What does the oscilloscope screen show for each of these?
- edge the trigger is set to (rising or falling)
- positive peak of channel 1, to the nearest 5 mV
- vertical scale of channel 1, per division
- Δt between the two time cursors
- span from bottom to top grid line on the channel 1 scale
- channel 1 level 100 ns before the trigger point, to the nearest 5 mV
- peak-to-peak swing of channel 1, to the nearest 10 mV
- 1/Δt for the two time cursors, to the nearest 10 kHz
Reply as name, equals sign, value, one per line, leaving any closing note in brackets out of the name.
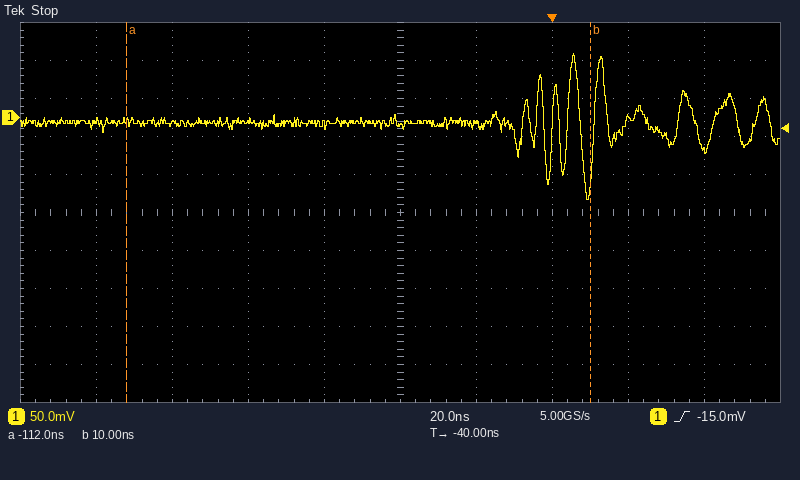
edge the trigger is set to = rising
positive peak of channel 1, to the nearest 5 mV = 85 mV
vertical scale of channel 1, per division = 50 mV
Δt between the two time cursors = 122 ns
span from bottom to top grid line on the channel 1 scale = 500 mV
channel 1 level 100 ns before the trigger point, to the nearest 5 mV = -10 mV
peak-to-peak swing of channel 1, to the nearest 10 mV = 190 mV
1/Δt for the two time cursors, to the nearest 10 kHz = 8.20 MHz
